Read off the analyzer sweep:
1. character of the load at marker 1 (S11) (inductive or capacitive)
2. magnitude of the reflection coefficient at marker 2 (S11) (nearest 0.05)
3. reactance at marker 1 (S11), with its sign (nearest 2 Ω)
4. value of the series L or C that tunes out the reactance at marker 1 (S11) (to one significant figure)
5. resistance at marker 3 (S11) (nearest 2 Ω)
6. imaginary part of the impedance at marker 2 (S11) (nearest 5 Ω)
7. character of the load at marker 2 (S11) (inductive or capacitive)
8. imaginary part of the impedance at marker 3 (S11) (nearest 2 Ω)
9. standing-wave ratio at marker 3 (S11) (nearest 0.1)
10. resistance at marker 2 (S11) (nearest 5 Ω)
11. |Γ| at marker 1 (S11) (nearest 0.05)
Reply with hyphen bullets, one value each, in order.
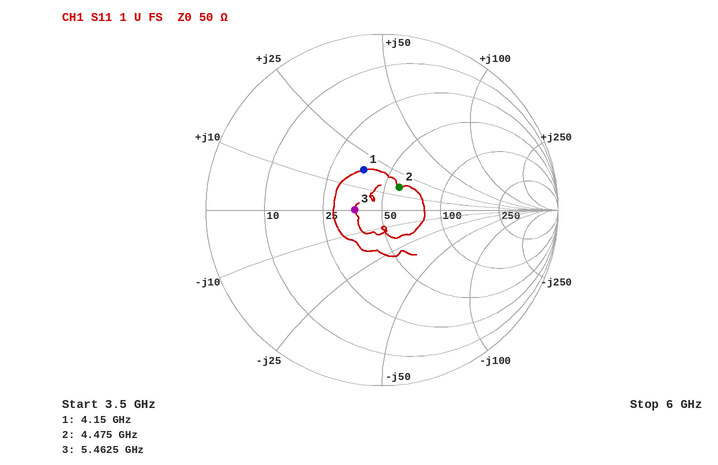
- inductive
- 0.15
- +18 Ω
- 2 pF
- 36 Ω
- +15 Ω
- inductive
- 0 Ω
- 1.4
- 60 Ω
- 0.25
